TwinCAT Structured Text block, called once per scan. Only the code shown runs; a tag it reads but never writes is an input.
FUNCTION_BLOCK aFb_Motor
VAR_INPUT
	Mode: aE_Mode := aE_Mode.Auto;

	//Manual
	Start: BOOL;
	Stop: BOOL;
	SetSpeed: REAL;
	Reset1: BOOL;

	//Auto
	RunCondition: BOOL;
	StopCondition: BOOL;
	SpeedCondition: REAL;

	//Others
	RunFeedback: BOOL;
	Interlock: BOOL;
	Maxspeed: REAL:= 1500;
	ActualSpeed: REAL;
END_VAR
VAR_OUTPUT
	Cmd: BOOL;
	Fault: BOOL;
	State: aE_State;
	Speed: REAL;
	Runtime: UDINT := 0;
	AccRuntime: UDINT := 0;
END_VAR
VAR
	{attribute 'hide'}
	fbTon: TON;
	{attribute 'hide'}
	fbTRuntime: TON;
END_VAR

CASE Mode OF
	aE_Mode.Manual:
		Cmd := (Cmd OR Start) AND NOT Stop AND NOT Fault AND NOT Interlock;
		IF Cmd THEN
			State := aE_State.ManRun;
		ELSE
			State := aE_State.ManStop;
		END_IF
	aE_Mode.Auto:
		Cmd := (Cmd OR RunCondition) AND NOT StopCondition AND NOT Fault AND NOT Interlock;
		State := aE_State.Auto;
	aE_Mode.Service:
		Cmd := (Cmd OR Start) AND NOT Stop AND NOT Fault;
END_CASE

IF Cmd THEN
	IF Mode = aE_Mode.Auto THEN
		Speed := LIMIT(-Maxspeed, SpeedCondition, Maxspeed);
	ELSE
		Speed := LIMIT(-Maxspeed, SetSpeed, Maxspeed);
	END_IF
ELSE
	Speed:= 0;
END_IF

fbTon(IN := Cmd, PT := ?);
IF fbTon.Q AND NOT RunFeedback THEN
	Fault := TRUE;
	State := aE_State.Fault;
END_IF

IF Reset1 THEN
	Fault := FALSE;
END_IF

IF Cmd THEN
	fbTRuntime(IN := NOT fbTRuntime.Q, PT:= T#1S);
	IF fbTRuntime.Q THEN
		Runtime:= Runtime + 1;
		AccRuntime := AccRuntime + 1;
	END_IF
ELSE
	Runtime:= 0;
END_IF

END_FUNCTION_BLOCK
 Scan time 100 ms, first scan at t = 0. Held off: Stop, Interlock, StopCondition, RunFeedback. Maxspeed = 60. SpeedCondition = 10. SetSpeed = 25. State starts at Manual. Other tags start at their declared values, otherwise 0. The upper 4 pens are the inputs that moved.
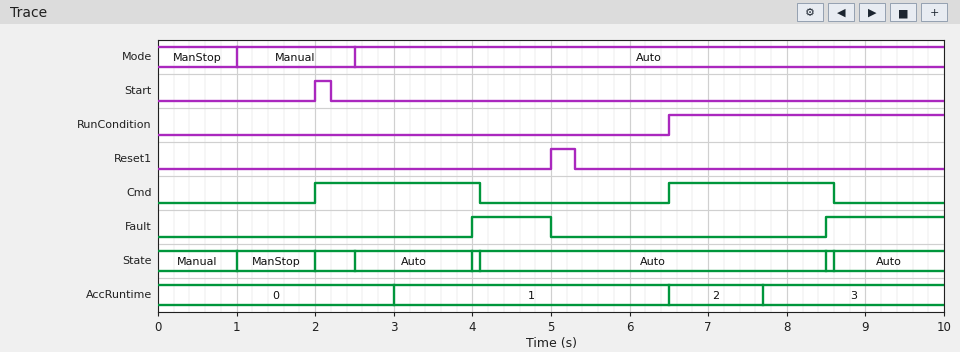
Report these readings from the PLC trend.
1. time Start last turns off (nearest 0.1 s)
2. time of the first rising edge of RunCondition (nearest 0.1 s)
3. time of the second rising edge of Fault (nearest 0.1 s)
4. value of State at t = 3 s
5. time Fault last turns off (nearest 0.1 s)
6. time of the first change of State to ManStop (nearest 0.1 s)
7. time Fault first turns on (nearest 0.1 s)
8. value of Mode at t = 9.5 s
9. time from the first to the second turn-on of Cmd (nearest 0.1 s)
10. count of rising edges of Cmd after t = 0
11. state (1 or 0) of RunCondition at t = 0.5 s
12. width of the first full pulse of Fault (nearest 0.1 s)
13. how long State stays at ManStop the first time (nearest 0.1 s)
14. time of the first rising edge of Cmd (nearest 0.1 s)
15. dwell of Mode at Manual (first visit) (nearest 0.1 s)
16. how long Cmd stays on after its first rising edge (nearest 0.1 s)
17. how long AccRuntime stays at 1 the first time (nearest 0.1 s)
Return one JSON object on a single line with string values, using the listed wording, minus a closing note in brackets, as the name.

{"time Start last turns off": "2.2 s", "time of the first rising edge of RunCondition": "6.5 s", "time of the second rising edge of Fault": "8.5 s", "value of State at t = 3 s": "Auto", "time Fault last turns off": "5.0 s", "time of the first change of State to ManStop": "1.0 s", "time Fault first turns on": "4.0 s", "value of Mode at t = 9.5 s": "Auto", "time from the first to the second turn-on of Cmd": "4.5 s", "count of rising edges of Cmd after t = 0": "2", "state (1 or 0) of RunCondition at t = 0.5 s": "0", "width of the first full pulse of Fault": "1.0 s", "how long State stays at ManStop the first time": "1.0 s", "time of the first rising edge of Cmd": "2.0 s", "dwell of Mode at Manual (first visit)": "1.5 s", "how long Cmd stays on after its first rising edge": "2.1 s", "how long AccRuntime stays at 1 the first time": "3.5 s"}
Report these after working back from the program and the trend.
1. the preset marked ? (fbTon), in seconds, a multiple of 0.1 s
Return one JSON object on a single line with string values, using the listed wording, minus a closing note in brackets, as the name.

{"the preset marked ? (fbTon), in seconds, a multiple of 0.1 s": "2.0 s"}
